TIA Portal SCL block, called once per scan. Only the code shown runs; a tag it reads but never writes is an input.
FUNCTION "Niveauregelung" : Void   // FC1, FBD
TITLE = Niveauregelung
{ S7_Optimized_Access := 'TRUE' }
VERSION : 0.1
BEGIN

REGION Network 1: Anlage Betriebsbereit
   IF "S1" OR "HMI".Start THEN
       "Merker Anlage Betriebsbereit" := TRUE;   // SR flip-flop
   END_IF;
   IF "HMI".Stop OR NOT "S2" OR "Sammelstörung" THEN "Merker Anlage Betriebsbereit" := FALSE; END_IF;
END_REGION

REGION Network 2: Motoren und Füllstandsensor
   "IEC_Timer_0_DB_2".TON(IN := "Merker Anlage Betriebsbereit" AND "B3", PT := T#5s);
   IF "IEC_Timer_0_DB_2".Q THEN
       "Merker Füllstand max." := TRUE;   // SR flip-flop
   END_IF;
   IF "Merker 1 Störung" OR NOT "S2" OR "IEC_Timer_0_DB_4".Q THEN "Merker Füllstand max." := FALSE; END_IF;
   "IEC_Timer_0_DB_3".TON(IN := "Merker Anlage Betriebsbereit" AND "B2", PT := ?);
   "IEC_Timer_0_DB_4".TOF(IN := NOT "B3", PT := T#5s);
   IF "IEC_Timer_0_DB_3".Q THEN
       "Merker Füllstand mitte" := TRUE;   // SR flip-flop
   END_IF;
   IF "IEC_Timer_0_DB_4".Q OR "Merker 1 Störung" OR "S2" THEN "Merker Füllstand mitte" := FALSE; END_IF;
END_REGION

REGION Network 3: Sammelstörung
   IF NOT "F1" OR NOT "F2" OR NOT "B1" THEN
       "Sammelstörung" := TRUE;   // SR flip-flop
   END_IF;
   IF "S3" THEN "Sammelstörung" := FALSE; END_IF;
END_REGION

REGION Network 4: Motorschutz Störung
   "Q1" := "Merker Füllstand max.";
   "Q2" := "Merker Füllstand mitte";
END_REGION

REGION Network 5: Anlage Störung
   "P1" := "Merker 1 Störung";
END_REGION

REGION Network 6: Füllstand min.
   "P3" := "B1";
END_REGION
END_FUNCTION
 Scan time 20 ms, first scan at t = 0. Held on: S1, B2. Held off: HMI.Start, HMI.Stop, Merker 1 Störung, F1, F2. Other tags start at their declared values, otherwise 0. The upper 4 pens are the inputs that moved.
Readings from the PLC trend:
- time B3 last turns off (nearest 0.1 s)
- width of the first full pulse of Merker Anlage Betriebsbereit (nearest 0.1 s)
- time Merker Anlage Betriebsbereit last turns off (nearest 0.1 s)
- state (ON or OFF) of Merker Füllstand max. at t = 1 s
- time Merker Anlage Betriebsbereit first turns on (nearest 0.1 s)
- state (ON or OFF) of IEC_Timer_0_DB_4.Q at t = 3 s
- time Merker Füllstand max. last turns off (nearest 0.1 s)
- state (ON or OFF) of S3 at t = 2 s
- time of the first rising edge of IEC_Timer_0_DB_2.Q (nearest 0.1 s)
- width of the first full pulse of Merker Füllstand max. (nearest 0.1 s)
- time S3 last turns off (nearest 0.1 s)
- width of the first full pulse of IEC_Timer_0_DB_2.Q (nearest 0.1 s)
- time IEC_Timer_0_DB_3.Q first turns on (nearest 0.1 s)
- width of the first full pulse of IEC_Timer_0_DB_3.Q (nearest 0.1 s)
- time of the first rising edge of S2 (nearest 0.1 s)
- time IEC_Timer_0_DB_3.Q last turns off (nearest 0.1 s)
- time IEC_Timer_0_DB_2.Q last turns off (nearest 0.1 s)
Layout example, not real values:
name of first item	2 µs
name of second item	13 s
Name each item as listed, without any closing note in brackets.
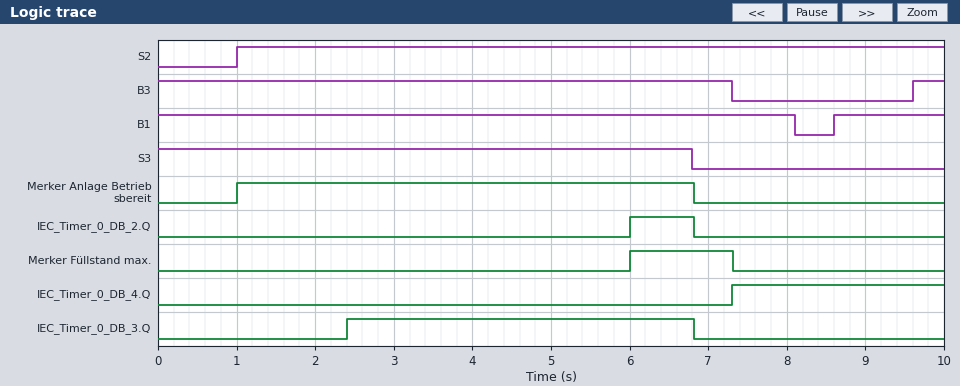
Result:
time B3 last turns off	7.3 s
width of the first full pulse of Merker Anlage Betriebsbereit	5.8 s
time Merker Anlage Betriebsbereit last turns off	6.8 s
state (ON or OFF) of Merker Füllstand max. at t = 1 s	OFF
time Merker Anlage Betriebsbereit first turns on	1.0 s
state (ON or OFF) of IEC_Timer_0_DB_4.Q at t = 3 s	OFF
time Merker Füllstand max. last turns off	7.3 s
state (ON or OFF) of S3 at t = 2 s	ON
time of the first rising edge of IEC_Timer_0_DB_2.Q	6.0 s
width of the first full pulse of Merker Füllstand max.	1.3 s
time S3 last turns off	6.8 s
width of the first full pulse of IEC_Timer_0_DB_2.Q	0.8 s
time IEC_Timer_0_DB_3.Q first turns on	2.4 s
width of the first full pulse of IEC_Timer_0_DB_3.Q	4.4 s
time of the first rising edge of S2	1.0 s
time IEC_Timer_0_DB_3.Q last turns off	6.8 s
time IEC_Timer_0_DB_2.Q last turns off	6.8 s
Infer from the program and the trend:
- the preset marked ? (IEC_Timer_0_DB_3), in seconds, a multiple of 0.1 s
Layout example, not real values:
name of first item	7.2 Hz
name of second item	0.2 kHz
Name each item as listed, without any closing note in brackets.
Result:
the preset marked ? (IEC_Timer_0_DB_3), in seconds, a multiple of 0.1 s	1.4 s
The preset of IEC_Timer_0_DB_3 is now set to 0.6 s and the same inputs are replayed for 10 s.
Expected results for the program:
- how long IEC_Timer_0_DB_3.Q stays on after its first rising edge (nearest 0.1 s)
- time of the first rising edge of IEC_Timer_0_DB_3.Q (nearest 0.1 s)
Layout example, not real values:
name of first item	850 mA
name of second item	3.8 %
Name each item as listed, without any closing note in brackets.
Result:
how long IEC_Timer_0_DB_3.Q stays on after its first rising edge	5.2 s
time of the first rising edge of IEC_Timer_0_DB_3.Q	1.6 s
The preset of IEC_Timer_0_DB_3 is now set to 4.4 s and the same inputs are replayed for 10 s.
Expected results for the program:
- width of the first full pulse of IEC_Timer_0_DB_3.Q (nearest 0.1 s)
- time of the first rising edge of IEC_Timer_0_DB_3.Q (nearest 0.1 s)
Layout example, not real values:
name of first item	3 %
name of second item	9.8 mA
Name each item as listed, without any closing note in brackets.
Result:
width of the first full pulse of IEC_Timer_0_DB_3.Q	1.4 s
time of the first rising edge of IEC_Timer_0_DB_3.Q	5.4 s
